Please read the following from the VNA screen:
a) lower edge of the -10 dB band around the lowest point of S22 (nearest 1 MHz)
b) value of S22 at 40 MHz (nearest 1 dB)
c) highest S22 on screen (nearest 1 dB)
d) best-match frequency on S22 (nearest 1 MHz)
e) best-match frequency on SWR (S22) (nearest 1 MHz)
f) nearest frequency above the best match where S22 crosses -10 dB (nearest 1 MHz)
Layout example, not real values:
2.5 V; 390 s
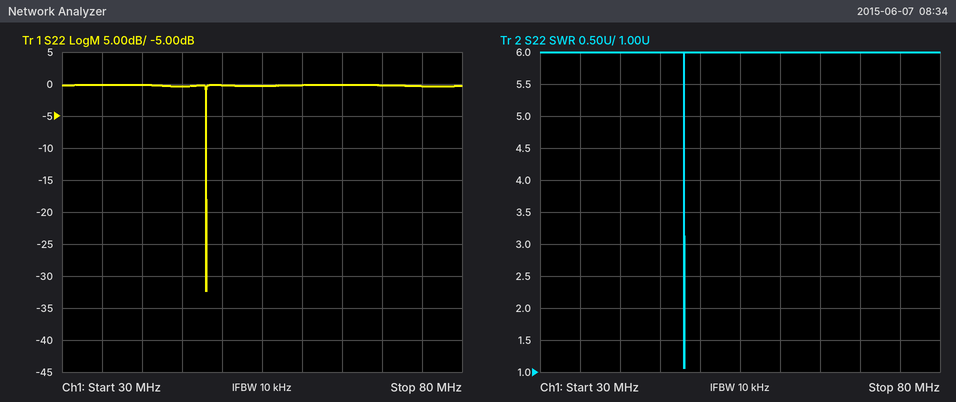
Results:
48 MHz; 0 dB; 0 dB; 48 MHz; 48 MHz; 48 MHz
